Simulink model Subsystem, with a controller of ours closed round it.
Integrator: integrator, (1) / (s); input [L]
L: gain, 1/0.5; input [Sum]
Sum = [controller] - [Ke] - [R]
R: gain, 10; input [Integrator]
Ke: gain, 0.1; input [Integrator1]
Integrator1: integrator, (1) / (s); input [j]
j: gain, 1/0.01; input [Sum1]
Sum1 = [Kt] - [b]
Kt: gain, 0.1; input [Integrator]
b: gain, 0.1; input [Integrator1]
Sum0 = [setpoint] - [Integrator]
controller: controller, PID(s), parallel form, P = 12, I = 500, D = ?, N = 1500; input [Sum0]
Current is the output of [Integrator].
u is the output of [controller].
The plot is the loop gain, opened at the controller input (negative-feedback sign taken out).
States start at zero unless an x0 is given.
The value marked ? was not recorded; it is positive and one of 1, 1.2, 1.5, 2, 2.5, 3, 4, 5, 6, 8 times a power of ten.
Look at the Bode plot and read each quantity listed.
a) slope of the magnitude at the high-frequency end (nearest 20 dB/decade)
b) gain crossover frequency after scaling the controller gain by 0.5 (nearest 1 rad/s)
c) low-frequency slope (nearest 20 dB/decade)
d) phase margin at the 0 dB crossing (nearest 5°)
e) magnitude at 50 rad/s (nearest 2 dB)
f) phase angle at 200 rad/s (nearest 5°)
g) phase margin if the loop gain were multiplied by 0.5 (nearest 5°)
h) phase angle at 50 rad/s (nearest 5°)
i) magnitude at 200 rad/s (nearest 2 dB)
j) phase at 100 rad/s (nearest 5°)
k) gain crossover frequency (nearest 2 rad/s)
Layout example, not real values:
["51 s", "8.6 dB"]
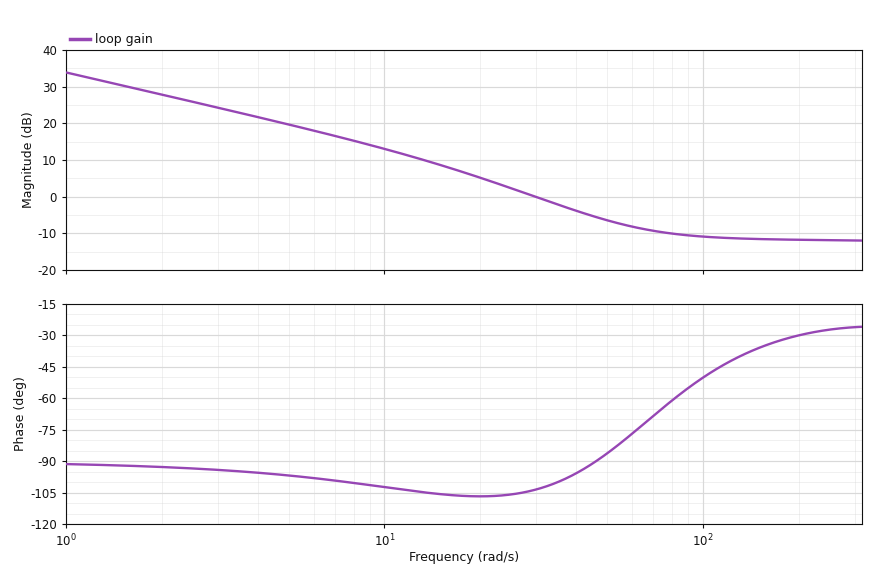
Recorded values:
["0 dB/decade", "19 rad/s", "-20 dB/decade", "75°", "-6 dB", "-30°", "75°", "-85°", "-12 dB", "-50°", "30 rad/s"]
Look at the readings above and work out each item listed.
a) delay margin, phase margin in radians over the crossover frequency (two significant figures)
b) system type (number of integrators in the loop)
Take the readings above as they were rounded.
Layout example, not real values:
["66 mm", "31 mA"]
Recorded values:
["0.044 s", "1"]
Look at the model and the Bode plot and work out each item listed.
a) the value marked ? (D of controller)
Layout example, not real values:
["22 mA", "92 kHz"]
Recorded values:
["0.12"]
